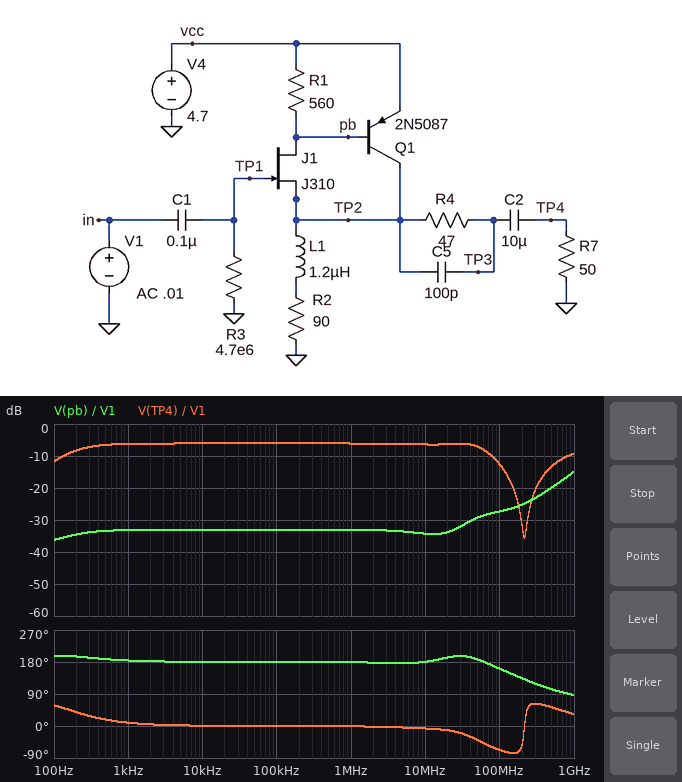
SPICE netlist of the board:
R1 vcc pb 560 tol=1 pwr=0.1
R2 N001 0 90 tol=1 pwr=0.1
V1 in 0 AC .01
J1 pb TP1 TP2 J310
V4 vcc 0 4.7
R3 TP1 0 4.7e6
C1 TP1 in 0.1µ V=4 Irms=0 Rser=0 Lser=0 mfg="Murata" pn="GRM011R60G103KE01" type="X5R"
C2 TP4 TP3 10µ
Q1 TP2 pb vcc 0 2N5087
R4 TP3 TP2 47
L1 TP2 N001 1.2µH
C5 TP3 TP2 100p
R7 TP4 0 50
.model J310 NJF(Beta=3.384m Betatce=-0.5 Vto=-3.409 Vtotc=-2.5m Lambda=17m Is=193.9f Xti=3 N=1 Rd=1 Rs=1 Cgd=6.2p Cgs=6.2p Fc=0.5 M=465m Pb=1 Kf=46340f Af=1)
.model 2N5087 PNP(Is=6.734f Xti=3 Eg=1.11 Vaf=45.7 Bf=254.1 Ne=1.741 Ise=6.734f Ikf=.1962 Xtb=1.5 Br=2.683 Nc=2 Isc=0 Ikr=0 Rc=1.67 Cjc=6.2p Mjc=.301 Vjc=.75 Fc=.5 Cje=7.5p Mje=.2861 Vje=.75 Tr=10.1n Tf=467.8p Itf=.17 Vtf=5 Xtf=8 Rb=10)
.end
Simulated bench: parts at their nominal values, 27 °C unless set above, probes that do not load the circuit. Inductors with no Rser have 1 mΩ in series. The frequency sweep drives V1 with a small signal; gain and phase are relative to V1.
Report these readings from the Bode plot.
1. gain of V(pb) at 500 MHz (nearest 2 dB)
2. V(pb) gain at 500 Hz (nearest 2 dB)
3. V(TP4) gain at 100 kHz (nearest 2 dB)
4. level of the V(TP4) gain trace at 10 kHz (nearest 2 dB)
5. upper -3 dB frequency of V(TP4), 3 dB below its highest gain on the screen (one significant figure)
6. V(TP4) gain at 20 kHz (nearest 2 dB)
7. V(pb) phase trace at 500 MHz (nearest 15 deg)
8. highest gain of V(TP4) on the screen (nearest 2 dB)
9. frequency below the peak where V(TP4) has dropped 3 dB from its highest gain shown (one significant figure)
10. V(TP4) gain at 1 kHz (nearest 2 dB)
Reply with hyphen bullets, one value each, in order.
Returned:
- -20 dB
- -34 dB
- -6 dB
- -6 dB
- 70 MHz
- -6 dB
- 105 deg
- -6 dB
- 200 Hz
- -6 dB
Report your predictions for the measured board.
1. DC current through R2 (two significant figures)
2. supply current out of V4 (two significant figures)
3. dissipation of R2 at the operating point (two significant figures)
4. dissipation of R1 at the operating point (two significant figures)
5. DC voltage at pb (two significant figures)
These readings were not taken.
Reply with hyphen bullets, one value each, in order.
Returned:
- 31 mA
- 31 mA
- 84 mW
- 1.0 mW
- 3.9 V
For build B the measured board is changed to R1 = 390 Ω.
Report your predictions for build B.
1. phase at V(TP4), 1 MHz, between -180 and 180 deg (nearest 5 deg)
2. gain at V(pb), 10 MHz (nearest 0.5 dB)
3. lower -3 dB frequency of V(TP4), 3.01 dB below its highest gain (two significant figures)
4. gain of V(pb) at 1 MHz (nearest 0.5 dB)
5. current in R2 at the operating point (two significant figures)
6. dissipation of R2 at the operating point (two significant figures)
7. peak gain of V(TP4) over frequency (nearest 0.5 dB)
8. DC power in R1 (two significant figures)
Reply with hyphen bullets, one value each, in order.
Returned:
- 0 deg
- -34.0 dB
- 180 Hz
- -32.5 dB
- 29 mA
- 77 mW
- -5.5 dB
- 1.5 mW
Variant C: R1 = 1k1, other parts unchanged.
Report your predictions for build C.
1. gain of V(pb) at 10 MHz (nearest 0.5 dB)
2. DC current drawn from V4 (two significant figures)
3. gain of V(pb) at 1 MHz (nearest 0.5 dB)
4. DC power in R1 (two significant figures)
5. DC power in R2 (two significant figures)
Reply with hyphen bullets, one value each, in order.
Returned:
- -35.0 dB
- 32 mA
- -33.5 dB
- 520 µW
- 95 mW
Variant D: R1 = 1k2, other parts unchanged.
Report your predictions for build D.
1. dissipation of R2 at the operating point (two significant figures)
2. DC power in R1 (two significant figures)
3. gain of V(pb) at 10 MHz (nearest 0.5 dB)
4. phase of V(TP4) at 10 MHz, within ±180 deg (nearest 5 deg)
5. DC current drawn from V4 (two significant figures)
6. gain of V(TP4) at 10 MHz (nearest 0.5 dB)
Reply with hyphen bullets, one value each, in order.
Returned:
- 96 mW
- 480 µW
- -35.0 dB
- -15 deg
- 33 mA
- -7.0 dB
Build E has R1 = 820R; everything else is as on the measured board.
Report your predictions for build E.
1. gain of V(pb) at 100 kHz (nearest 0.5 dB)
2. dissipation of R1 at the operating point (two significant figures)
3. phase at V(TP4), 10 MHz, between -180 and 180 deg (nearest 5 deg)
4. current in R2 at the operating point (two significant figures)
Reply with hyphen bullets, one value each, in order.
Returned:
- -33.5 dB
- 700 µW
- -10 deg
- 32 mA
